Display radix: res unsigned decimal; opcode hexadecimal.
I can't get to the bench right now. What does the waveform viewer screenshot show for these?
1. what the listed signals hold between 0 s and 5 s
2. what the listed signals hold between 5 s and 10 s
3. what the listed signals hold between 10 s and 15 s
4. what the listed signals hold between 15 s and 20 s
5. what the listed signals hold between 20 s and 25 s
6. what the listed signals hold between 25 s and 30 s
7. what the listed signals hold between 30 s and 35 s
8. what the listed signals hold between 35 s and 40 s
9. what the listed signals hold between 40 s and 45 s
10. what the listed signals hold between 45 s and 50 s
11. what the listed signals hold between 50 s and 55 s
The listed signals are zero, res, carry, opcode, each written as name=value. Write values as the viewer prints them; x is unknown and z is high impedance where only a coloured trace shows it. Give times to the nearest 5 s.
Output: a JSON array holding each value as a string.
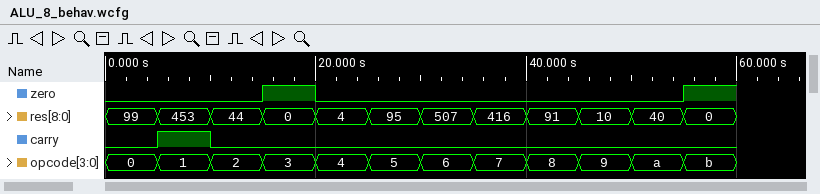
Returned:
["zero=0, res=99, carry=0, opcode=0", "zero=0, res=453, carry=1, opcode=1", "zero=0, res=44, carry=0, opcode=2", "zero=1, res=0, carry=0, opcode=3", "zero=0, res=4, carry=0, opcode=4", "zero=0, res=95, carry=0, opcode=5", "zero=0, res=507, carry=0, opcode=6", "zero=0, res=416, carry=0, opcode=7", "zero=0, res=91, carry=0, opcode=8", "zero=0, res=10, carry=0, opcode=9", "zero=0, res=40, carry=0, opcode=a"]
